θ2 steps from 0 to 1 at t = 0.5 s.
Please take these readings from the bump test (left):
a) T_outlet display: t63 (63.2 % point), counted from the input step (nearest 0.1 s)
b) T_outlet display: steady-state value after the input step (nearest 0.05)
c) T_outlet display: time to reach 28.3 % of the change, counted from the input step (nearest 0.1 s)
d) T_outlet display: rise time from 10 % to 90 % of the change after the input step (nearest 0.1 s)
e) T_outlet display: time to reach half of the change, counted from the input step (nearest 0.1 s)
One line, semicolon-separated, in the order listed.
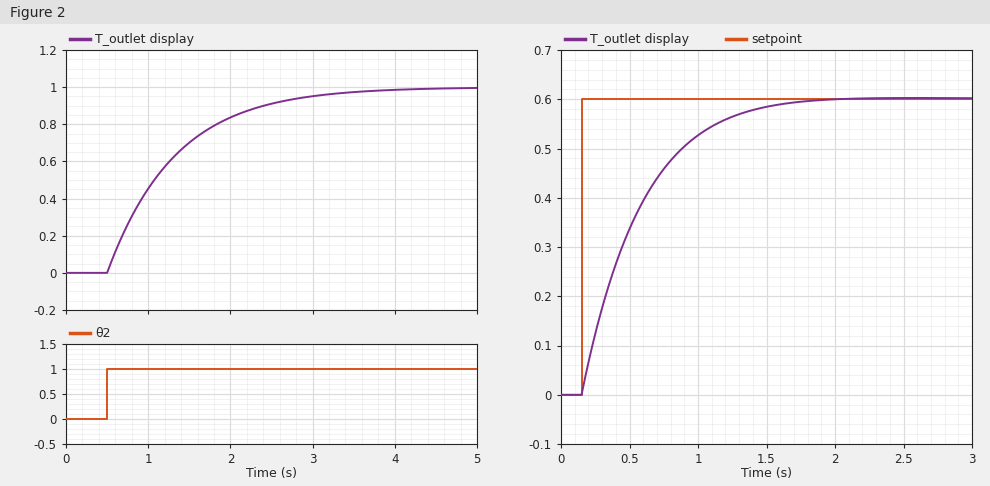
0.8 s; 1.00; 0.3 s; 1.8 s; 0.6 s
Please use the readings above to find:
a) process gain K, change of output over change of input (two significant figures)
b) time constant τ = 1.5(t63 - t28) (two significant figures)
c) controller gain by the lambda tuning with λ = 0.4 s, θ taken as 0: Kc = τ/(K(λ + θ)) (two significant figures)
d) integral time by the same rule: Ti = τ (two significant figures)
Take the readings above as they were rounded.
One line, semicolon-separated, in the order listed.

1.0; 0.75 s; 1.9; 0.75 s
